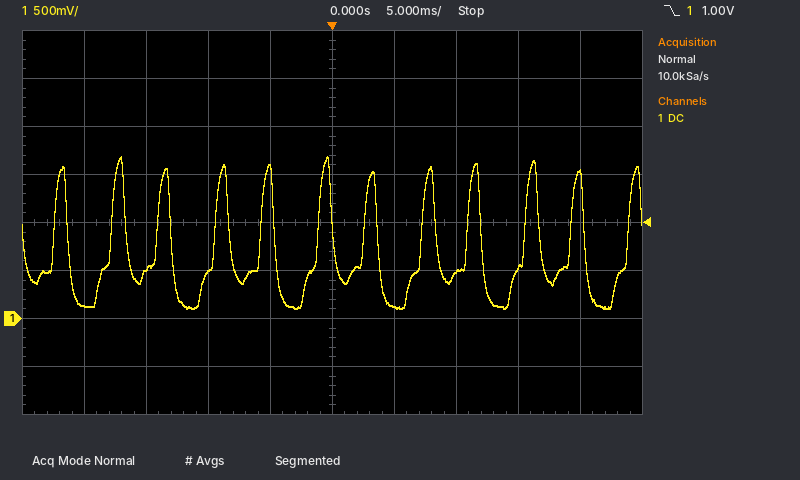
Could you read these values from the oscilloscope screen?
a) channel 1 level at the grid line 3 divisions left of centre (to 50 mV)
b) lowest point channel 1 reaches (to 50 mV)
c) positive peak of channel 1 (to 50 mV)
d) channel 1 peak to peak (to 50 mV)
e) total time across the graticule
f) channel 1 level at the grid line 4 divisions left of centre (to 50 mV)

500 mV
100 mV
1.70 V
1.60 V
50 ms
150 mV
